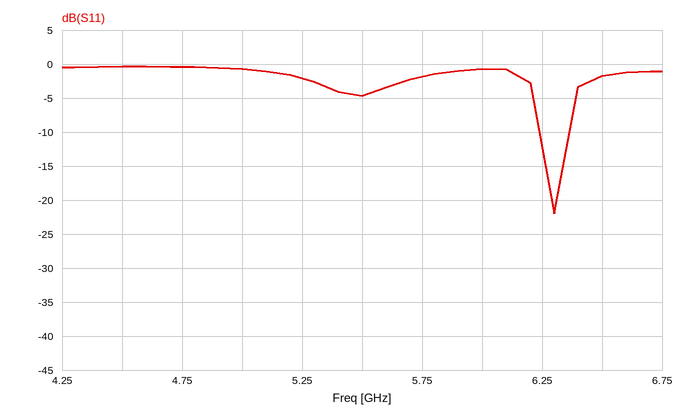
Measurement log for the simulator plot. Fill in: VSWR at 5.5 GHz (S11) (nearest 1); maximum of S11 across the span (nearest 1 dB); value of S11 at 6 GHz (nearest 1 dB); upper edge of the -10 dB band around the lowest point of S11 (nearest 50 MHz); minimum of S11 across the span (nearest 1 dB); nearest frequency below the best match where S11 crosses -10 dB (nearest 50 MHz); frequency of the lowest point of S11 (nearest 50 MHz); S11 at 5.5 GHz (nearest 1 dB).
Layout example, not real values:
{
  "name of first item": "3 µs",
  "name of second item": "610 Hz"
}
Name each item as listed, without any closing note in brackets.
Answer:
{
  "VSWR at 5.5 GHz (S11)": "4",
  "maximum of S11 across the span": "0 dB",
  "value of S11 at 6 GHz": "-1 dB",
  "upper edge of the -10 dB band around the lowest point of S11": "6.35 GHz",
  "minimum of S11 across the span": "-22 dB",
  "nearest frequency below the best match where S11 crosses -10 dB": "6.25 GHz",
  "frequency of the lowest point of S11": "6.30 GHz",
  "S11 at 5.5 GHz": "-5 dB"
}
